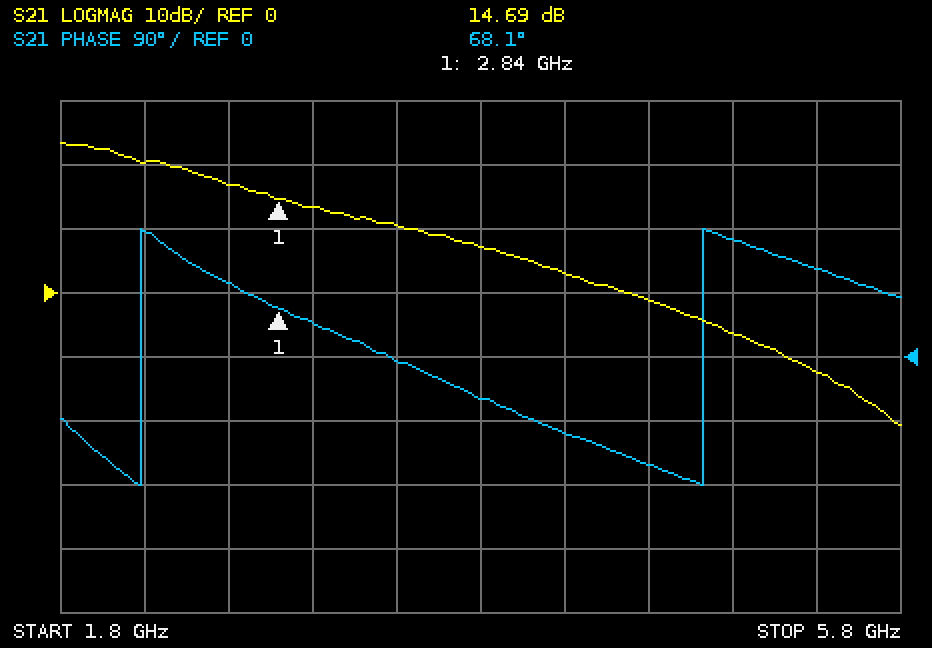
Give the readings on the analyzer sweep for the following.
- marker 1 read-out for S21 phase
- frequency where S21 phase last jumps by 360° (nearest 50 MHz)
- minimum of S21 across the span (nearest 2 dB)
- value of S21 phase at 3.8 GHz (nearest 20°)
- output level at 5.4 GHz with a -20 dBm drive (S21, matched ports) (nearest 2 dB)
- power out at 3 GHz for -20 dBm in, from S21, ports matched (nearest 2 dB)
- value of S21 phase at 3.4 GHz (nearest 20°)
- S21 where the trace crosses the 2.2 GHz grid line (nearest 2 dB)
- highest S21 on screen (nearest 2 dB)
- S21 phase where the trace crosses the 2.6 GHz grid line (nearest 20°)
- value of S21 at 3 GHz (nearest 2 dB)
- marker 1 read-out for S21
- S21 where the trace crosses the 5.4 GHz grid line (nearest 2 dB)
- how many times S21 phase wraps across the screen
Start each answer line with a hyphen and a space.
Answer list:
- 68.1°
- 4.85 GHz
- -20 dB
- -60°
- -32 dBm
- -6 dBm
- 0°
- 20 dB
- 24 dB
- 100°
- 14 dB
- 14.69 dB
- -12 dB
- 2
